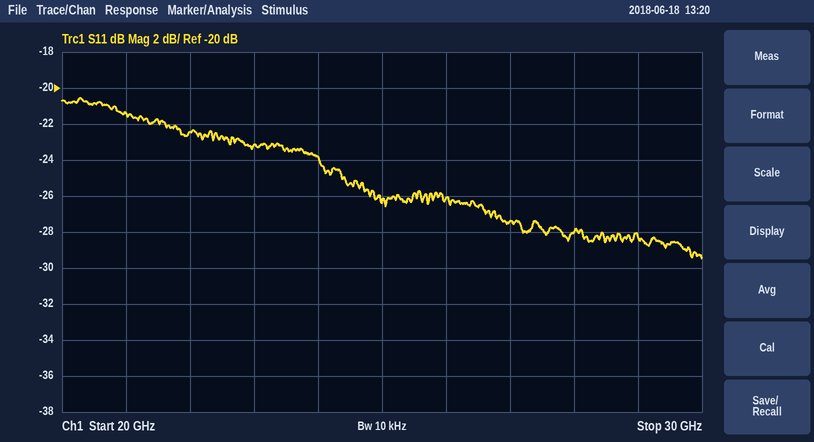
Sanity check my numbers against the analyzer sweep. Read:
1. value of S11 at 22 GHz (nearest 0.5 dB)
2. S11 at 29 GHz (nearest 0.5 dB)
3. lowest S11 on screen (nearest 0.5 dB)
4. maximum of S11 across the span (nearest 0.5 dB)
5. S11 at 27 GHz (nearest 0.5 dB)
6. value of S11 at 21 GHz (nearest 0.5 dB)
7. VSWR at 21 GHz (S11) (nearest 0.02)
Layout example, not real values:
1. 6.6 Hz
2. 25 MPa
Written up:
1. -22.5 dB
2. -28.5 dB
3. -29.5 dB
4. -20.5 dB
5. -27.5 dB
6. -21.5 dB
7. 1.18
